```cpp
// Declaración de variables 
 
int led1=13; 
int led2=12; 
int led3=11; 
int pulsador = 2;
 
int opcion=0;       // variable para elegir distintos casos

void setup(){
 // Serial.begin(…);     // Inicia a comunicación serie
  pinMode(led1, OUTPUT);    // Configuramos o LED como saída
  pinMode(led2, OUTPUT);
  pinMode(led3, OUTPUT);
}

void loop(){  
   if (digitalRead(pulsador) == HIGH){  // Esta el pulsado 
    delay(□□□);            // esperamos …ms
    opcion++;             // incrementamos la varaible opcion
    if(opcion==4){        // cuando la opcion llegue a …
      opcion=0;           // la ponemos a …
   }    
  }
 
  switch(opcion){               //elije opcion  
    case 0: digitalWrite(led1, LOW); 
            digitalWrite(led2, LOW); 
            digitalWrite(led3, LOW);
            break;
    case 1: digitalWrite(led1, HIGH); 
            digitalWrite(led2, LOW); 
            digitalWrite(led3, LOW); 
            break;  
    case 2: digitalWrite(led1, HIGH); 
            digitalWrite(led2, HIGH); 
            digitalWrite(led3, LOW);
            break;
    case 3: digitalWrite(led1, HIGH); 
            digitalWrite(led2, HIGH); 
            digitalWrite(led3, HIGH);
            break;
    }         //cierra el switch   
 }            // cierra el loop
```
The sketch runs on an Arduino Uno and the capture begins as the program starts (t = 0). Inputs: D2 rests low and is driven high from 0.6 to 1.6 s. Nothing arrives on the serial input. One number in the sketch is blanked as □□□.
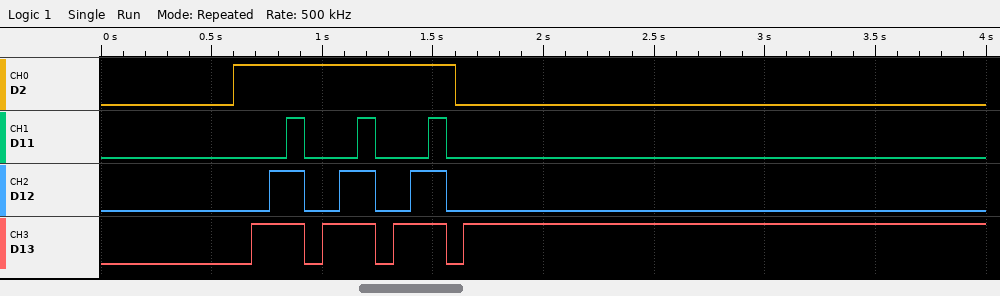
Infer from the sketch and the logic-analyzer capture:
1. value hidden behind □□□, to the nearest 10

80
